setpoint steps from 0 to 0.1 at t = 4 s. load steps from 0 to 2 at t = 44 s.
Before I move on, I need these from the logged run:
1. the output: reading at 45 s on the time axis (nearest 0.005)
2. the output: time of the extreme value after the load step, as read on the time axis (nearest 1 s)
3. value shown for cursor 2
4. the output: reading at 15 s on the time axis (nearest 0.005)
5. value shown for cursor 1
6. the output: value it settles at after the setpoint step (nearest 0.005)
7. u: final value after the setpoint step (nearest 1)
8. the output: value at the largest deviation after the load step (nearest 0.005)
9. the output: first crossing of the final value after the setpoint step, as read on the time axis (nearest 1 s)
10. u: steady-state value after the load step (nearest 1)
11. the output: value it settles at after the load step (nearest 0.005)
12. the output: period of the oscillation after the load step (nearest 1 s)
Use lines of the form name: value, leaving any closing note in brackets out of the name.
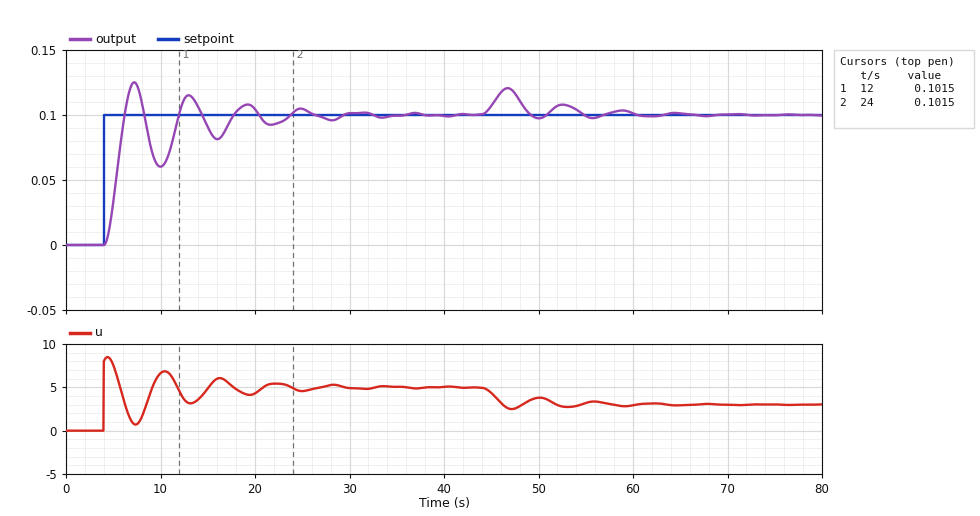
the output: reading at 45 s on the time axis: 0.105
the output: time of the extreme value after the load step, as read on the time axis: 47 s
value shown for cursor 2: 0.1015
the output: reading at 15 s on the time axis: 0.090
value shown for cursor 1: 0.1015
the output: value it settles at after the setpoint step: 0.100
u: final value after the setpoint step: 5
the output: value at the largest deviation after the load step: 0.120
the output: first crossing of the final value after the setpoint step, as read on the time axis: 6 s
u: steady-state value after the load step: 3
the output: value it settles at after the load step: 0.100
the output: period of the oscillation after the load step: 6 s
